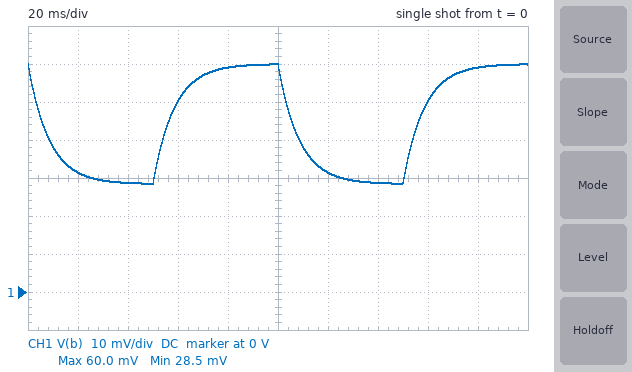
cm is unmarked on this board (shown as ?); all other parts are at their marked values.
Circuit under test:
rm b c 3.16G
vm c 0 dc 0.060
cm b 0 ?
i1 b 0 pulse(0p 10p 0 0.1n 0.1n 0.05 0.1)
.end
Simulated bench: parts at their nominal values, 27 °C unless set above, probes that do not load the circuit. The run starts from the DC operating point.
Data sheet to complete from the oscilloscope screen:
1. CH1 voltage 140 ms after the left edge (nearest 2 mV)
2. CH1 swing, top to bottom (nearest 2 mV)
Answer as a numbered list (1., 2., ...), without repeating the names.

1. 28 mV
2. 32 mV
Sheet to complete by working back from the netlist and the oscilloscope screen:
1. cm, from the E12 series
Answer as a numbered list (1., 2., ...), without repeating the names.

1. 2.7 pF
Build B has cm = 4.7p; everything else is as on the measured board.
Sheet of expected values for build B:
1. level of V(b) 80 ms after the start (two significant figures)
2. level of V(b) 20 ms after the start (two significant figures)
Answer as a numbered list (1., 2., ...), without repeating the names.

1. 56 mV
2. 37 mV
